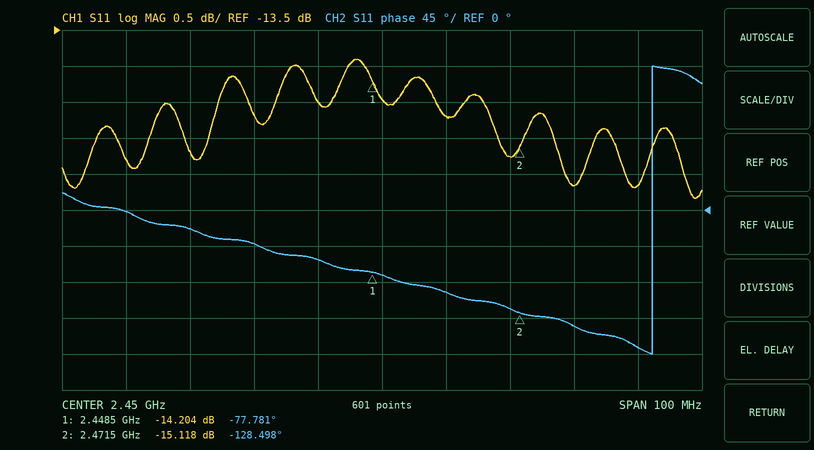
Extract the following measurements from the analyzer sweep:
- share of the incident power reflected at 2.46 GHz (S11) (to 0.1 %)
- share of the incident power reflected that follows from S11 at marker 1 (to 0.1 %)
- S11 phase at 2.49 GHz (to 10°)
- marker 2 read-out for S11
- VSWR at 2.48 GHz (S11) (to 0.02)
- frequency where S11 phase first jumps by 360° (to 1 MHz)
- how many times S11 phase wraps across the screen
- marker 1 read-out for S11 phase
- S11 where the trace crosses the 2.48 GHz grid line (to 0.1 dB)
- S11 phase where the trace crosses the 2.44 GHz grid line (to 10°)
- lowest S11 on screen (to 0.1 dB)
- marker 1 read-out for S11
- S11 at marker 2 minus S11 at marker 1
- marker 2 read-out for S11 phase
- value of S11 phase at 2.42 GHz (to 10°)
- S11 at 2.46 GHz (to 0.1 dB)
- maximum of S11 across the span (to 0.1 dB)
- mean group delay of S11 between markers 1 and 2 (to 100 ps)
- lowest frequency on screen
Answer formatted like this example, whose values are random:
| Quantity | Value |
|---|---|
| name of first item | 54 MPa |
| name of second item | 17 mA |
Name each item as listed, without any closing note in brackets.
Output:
| Quantity | Value |
|---|---|
| share of the incident power reflected at 2.46 GHz (S11) | 3.4 % |
| share of the incident power reflected that follows from S11 at marker 1 | 3.8 % |
| S11 phase at 2.49 GHz | -170° |
| marker 2 read-out for S11 | -15.118 dB |
| VSWR at 2.48 GHz (S11) | 1.40 |
| frequency where S11 phase first jumps by 360° | 2.492 GHz |
| how many times S11 phase wraps across the screen | 1 |
| marker 1 read-out for S11 phase | -77.781° |
| S11 where the trace crosses the 2.48 GHz grid line | -15.7 dB |
| S11 phase where the trace crosses the 2.44 GHz grid line | -60° |
| lowest S11 on screen | -15.8 dB |
| marker 1 read-out for S11 | -14.204 dB |
| S11 at marker 2 minus S11 at marker 1 | -0.914 dB |
| marker 2 read-out for S11 phase | -128.498° |
| value of S11 phase at 2.42 GHz | -20° |
| S11 at 2.46 GHz | -14.7 dB |
| maximum of S11 across the span | -13.9 dB |
| mean group delay of S11 between markers 1 and 2 | 6.1 ns |
| lowest frequency on screen | 2.4 GHz |
